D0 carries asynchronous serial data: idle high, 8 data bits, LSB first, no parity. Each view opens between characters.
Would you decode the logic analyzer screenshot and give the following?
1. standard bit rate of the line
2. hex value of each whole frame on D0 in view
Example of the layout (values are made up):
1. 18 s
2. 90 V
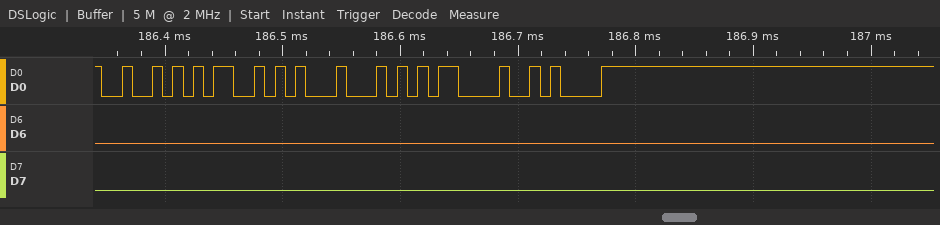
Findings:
1. 115200 baud
2. 52, 53, 44, 0D, 0A
